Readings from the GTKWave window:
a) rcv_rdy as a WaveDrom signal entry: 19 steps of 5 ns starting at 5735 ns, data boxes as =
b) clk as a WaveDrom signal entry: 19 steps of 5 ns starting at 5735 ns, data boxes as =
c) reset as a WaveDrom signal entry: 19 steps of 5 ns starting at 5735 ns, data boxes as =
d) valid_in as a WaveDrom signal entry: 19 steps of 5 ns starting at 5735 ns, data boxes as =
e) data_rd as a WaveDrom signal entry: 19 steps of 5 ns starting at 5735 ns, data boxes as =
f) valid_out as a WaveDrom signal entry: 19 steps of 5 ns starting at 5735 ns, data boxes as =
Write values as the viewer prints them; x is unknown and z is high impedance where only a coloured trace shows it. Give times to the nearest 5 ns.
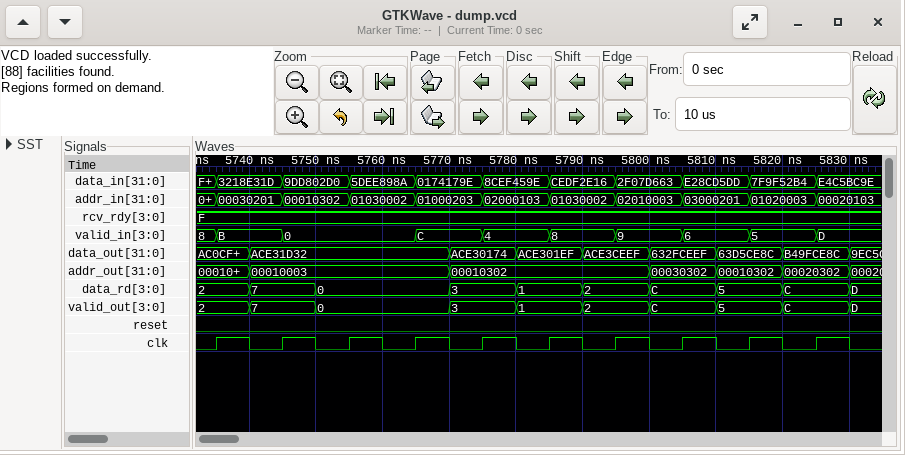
{name: 'rcv_rdy', wave: '=..................', data: 'F'}
{name: 'clk', wave: '1010101010101010101'}
{name: 'reset', wave: '0..................'}
{name: 'valid_in', wave: '=.=...=.=.=.=.=.=.=', data: 'B 0 C 4 8 9 6 5 D'}
{name: 'data_rd', wave: '==.=...=.=.=.=.=.=.', data: '2 7 0 3 1 2 C 5 C'}
{name: 'valid_out', wave: '==.=...=.=.=.=.=.=.', data: '2 7 0 3 1 2 C 5 C'}
